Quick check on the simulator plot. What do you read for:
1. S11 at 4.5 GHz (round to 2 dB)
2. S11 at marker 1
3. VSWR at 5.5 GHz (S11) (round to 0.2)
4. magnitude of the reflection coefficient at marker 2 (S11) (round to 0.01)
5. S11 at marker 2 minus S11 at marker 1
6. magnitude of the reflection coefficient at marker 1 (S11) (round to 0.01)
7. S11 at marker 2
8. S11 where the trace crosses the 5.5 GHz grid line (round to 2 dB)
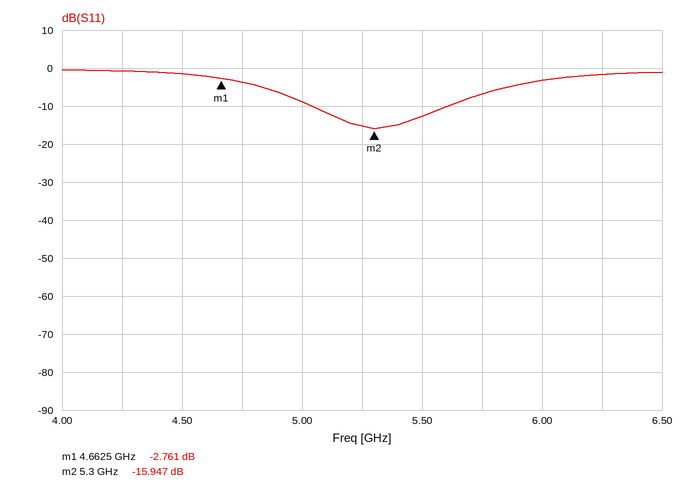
-2 dB
-2.761 dB
1.6
0.16
-13.186 dB
0.73
-15.947 dB
-12 dB
